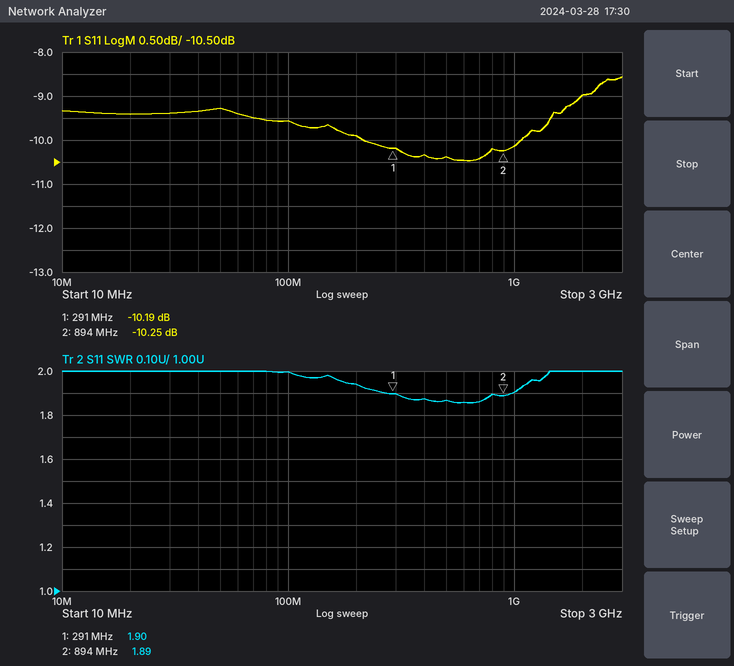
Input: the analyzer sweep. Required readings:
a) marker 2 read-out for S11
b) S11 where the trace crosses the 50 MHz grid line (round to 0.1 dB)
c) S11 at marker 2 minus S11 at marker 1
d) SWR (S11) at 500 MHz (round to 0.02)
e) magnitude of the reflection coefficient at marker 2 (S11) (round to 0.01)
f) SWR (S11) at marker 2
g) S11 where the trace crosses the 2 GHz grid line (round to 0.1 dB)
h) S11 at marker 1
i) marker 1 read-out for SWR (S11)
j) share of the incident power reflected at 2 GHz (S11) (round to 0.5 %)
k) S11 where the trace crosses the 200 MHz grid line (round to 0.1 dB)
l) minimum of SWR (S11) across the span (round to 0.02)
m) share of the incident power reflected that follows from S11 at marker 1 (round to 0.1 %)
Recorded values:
-10.25 dB
-9.3 dB
-0.06 dB
1.86
0.31
1.89
-9.0 dB
-10.19 dB
1.90
12.5 %
-9.9 dB
1.86
9.6 %
